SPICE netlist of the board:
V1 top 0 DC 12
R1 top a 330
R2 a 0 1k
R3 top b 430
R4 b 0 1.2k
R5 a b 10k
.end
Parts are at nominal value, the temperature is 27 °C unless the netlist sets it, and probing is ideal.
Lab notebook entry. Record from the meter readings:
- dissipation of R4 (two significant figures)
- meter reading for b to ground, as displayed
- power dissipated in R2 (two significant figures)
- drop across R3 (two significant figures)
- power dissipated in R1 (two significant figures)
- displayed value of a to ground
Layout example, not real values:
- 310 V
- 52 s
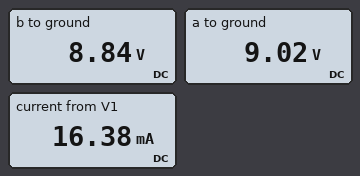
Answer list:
- 65 mW
- 8.84 V
- 81 mW
- 3.2 V
- 27 mW
- 9.02 V
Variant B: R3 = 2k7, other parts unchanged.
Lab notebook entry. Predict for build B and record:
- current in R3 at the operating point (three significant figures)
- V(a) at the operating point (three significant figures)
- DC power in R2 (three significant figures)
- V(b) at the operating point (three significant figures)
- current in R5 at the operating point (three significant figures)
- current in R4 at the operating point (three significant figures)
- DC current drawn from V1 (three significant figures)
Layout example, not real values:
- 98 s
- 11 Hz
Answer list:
- 2.93 mA
- 8.90 V
- 79.3 mW
- 4.09 V
- 481 µA
- 3.41 mA
- 12.3 mA
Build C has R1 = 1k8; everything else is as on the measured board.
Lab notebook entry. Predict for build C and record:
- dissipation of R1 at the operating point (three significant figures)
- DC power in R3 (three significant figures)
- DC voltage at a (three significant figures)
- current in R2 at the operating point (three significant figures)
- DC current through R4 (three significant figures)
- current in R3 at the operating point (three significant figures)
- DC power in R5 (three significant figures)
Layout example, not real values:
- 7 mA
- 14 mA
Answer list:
- 30.8 mW
- 25.3 mW
- 4.55 V
- 4.55 mA
- 7.25 mA
- 7.67 mA
- 1.72 mW
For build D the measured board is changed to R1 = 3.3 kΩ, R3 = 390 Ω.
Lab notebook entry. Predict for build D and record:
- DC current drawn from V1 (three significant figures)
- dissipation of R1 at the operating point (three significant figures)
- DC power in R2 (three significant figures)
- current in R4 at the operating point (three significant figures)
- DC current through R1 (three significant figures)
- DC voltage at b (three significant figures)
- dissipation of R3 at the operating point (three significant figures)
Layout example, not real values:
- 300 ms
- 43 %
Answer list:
- 10.6 mA
- 23.3 mW
- 10.4 mW
- 7.41 mA
- 2.66 mA
- 8.89 V
- 24.8 mW
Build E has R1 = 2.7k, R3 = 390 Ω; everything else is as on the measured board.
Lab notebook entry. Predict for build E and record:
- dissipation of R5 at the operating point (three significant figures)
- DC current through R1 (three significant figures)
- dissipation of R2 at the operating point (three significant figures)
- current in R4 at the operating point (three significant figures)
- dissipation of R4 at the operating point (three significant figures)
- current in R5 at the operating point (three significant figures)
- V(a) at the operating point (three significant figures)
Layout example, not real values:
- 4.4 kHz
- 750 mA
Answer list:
- 2.78 mW
- 3.10 mA
- 13.2 mW
- 7.42 mA
- 66.0 mW
- 527 µA
- 3.63 V
